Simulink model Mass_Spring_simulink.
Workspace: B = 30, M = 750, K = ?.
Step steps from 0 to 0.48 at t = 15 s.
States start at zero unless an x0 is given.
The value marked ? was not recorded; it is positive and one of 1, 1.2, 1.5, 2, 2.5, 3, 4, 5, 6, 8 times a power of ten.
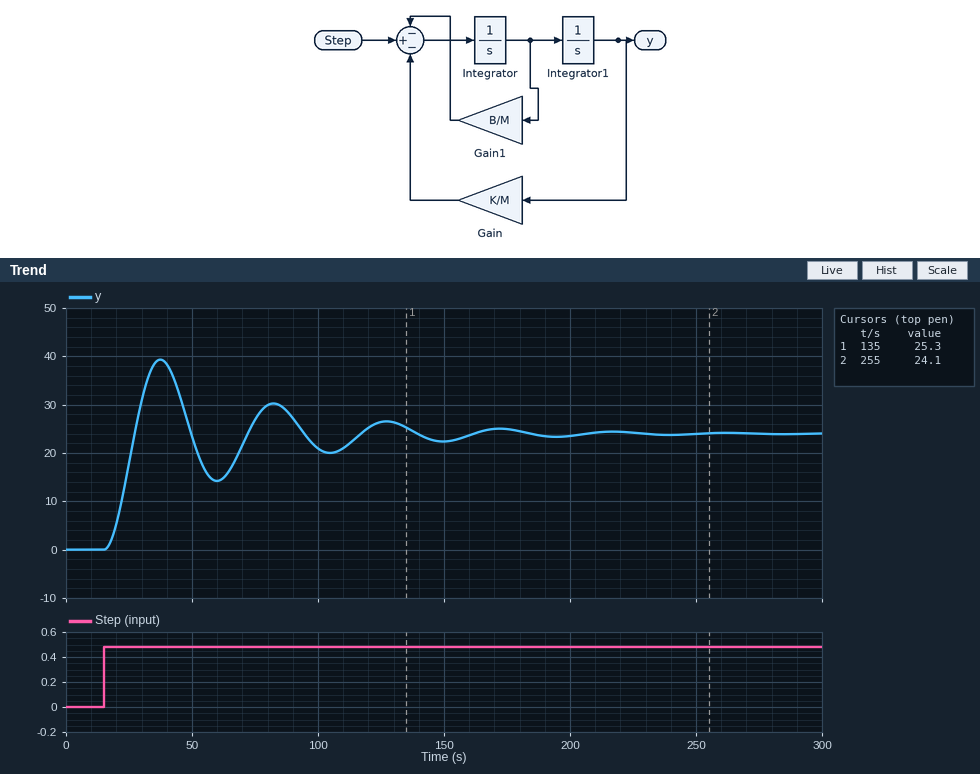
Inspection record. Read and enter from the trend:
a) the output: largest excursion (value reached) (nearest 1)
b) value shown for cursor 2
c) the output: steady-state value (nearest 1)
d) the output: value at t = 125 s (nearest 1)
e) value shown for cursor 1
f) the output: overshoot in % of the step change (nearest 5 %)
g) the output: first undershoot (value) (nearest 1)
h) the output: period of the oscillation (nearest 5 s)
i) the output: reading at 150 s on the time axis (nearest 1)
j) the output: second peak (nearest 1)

39
24.1
24
26
25.3
65 %
14
45 s
22
30
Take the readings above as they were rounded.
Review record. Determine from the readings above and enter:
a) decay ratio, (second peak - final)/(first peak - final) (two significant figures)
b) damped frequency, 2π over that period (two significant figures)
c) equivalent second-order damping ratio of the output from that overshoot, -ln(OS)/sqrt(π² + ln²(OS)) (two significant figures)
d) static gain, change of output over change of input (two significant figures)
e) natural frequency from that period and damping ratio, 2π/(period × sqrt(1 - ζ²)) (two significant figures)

0.40
0.14 rad/s
0.14
50
0.14 rad/s
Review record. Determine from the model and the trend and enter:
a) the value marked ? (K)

15
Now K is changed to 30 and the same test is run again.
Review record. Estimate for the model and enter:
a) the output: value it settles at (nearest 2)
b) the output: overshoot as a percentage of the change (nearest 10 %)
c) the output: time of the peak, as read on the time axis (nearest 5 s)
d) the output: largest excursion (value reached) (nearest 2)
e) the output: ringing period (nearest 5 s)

12
70 %
30 s
20
30 s
